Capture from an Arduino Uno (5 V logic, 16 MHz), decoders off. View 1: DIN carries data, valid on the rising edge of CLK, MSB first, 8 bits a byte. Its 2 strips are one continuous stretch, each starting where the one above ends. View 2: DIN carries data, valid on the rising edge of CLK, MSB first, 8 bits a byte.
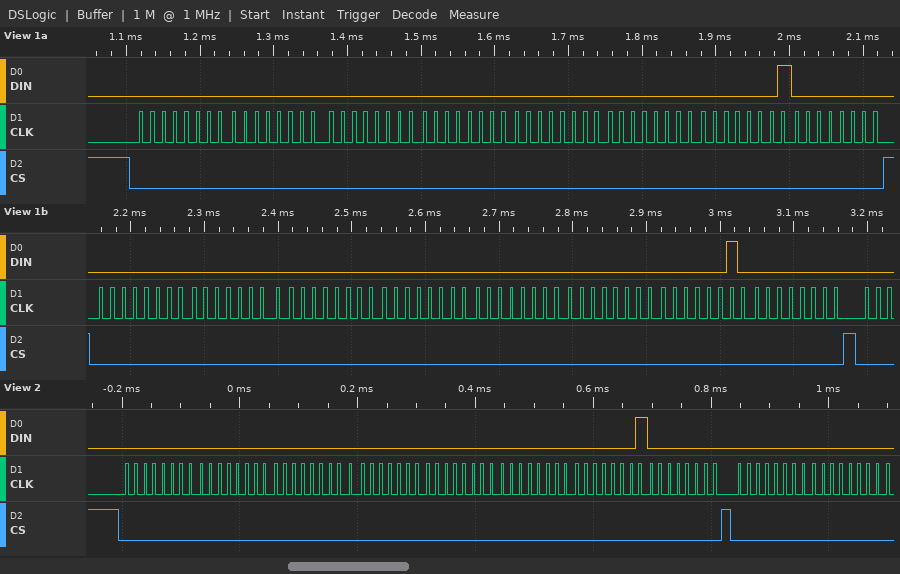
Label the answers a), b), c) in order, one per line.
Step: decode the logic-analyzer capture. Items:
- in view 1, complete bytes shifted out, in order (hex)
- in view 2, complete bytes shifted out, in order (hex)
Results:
a) 00 00 00 00 00 00 01 00 00 00 00 00 00 00 02 00
b) 00 00 00 00 00 00 01 00 00 00
